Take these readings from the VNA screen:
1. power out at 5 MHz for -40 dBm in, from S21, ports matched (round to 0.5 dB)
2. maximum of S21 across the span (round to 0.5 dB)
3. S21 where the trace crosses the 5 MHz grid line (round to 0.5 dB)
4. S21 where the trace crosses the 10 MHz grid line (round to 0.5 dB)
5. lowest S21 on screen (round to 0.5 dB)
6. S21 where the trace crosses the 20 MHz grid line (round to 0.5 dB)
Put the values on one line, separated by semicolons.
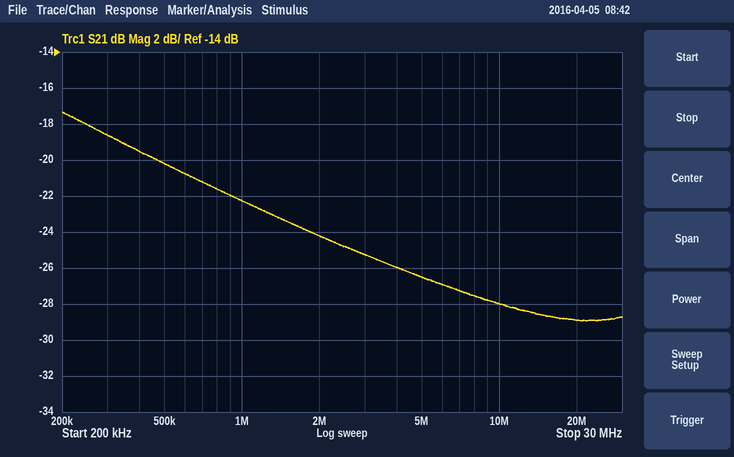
-66.5 dBm; -17.5 dB; -26.5 dB; -28.0 dB; -29.0 dB; -29.0 dB
